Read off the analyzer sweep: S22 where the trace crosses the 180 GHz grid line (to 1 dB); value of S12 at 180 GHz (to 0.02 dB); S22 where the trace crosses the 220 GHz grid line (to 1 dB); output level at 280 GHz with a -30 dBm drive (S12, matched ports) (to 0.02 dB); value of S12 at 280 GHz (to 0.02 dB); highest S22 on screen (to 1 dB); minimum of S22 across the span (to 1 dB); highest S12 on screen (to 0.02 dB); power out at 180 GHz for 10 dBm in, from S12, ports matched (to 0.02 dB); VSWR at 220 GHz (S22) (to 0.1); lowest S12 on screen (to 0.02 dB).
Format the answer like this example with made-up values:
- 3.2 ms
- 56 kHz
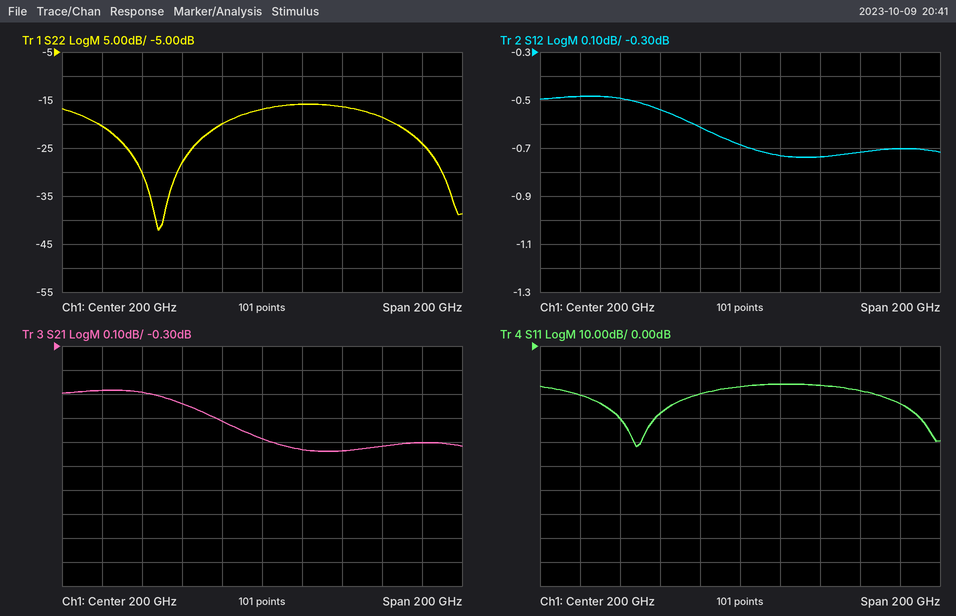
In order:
- -20 dB
- -0.62 dB
- -16 dB
- -30.70 dBm
- -0.70 dB
- -16 dB
- -42 dB
- -0.48 dB
- 9.38 dBm
- 1.4
- -0.74 dB
